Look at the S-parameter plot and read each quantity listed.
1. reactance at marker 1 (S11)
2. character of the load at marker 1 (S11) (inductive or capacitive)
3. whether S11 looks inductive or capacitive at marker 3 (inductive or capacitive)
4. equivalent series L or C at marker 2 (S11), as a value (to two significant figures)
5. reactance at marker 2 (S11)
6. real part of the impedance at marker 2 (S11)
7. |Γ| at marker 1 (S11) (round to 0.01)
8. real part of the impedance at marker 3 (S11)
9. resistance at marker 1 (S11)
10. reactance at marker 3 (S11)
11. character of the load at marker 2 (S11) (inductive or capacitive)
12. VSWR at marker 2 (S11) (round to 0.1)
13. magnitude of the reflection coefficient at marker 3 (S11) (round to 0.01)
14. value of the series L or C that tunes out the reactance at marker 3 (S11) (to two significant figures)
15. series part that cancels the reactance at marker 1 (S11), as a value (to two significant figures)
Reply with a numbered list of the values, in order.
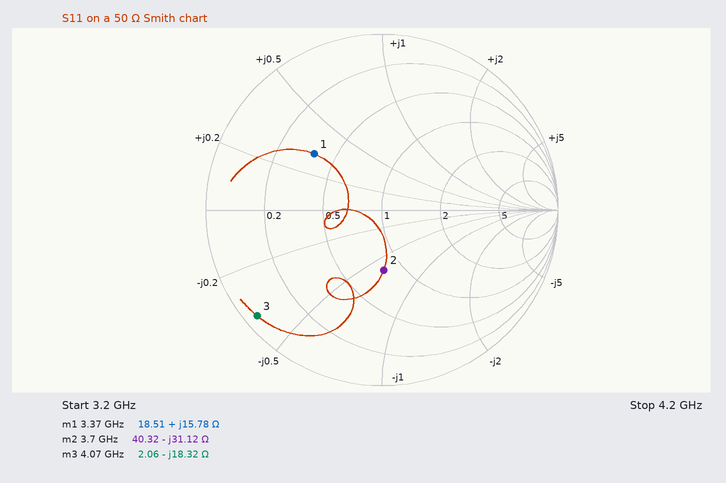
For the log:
1. +15.78 Ω
2. inductive
3. capacitive
4. 1.4 pF
5. -31.12 Ω
6. 40.32 Ω
7. 0.50
8. 2.06 Ω
9. 18.51 Ω
10. -18.32 Ω
11. capacitive
12. 2.0
13. 0.93
14. 720 pH
15. 3.0 pF
